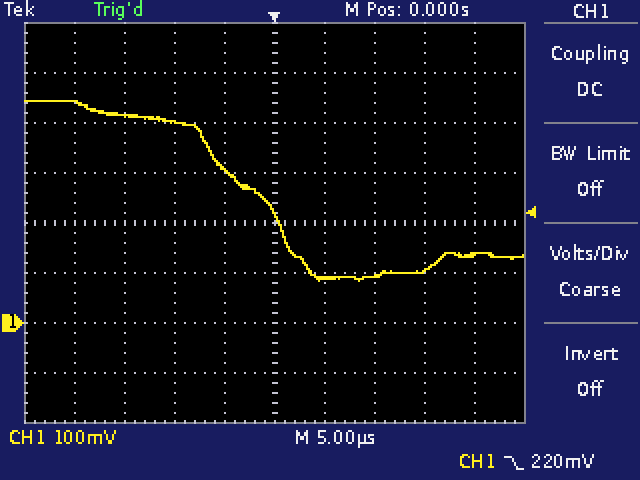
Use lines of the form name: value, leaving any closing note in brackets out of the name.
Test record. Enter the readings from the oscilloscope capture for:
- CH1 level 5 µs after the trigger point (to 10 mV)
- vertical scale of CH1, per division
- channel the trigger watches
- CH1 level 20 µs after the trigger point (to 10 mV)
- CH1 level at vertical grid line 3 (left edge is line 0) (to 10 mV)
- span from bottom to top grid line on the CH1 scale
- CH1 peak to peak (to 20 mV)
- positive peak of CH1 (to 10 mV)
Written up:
CH1 level 5 µs after the trigger point: 90 mV
vertical scale of CH1, per division: 100 mV
channel the trigger watches: CH1
CH1 level 20 µs after the trigger point: 140 mV
CH1 level at vertical grid line 3 (left edge is line 0): 400 mV
span from bottom to top grid line on the CH1 scale: 800 mV
CH1 peak to peak: 360 mV
positive peak of CH1: 440 mV
